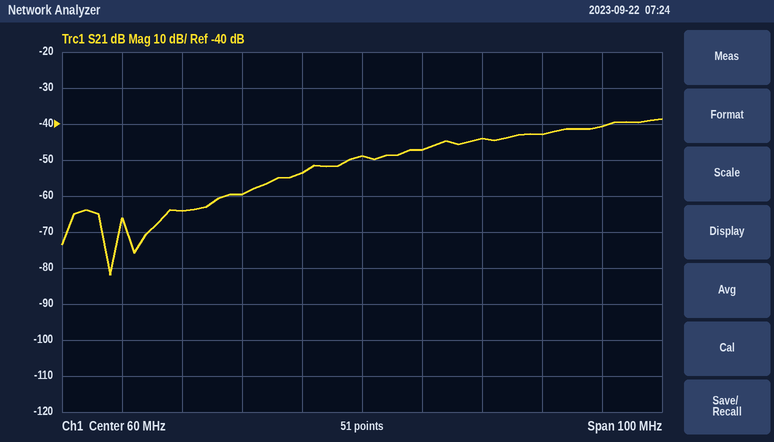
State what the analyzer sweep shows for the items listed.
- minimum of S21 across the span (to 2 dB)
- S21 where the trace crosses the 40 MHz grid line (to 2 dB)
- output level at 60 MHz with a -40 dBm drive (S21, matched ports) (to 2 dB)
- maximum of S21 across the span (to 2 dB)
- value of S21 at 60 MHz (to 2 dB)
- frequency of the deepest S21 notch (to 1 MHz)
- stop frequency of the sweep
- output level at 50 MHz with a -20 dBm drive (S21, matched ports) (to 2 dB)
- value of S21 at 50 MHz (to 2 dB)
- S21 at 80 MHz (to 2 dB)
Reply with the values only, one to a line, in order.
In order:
-82 dB
-60 dB
-88 dBm
-38 dB
-48 dB
18 MHz
110 MHz
-74 dBm
-54 dB
-44 dB
